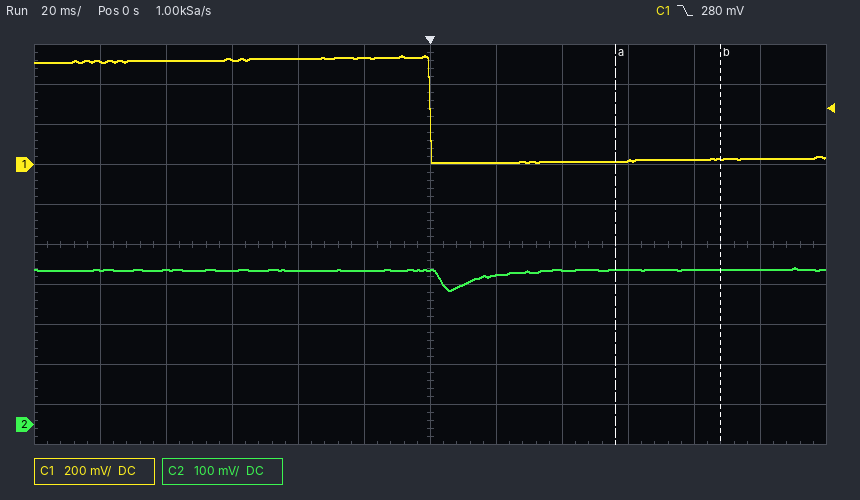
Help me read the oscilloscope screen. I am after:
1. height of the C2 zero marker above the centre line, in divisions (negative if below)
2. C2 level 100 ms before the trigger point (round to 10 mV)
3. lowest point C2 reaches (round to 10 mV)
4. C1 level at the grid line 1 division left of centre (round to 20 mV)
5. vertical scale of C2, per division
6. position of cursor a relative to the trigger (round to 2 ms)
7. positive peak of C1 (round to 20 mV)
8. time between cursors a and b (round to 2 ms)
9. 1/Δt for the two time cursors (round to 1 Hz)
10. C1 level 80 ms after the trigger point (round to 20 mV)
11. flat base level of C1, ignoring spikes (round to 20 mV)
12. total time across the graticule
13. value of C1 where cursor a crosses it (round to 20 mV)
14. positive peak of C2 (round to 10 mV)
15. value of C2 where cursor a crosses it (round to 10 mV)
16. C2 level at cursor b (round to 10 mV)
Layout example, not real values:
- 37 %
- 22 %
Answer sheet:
- -4.5 div
- 390 mV
- 340 mV
- 540 mV
- 100 mV
- +56 ms
- 540 mV
- 32 ms
- 31 Hz
- 20 mV
- 20 mV
- 240 ms
- 20 mV
- 390 mV
- 390 mV
- 390 mV
